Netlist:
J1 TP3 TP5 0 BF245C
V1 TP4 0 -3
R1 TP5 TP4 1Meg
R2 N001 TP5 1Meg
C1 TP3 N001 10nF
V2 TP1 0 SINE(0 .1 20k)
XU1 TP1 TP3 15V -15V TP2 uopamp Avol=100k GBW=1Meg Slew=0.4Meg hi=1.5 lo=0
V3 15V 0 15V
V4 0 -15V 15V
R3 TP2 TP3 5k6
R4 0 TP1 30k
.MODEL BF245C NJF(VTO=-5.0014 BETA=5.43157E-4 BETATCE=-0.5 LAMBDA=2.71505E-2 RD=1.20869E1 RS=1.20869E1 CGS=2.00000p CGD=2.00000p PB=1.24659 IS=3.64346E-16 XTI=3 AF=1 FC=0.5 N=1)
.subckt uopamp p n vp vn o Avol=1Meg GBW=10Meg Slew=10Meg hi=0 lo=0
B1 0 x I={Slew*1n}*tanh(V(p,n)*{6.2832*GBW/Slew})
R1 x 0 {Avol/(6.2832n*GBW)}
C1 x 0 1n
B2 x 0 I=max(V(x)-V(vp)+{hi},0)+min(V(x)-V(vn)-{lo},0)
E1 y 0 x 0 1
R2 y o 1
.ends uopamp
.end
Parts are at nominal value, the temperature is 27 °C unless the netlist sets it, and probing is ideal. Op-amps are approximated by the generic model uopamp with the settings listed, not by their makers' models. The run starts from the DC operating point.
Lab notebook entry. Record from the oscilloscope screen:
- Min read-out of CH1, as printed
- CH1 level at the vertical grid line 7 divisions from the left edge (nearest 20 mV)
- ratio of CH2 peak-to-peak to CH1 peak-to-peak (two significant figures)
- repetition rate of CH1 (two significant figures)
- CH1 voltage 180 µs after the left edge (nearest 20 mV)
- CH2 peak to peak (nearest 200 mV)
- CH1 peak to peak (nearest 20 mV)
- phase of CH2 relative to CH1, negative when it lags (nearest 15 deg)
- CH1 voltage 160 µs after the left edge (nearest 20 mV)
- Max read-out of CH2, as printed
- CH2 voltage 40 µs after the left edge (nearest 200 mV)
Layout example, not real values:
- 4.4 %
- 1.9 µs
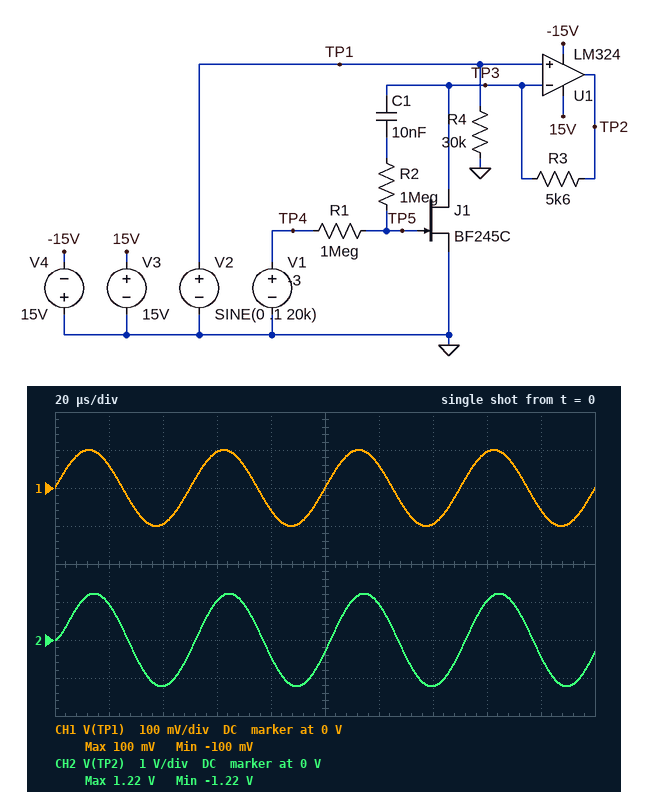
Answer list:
- -100 mV
- -100 mV
- 12
- 20 kHz
- -60 mV
- 2.4 V
- 200 mV
- -15 deg
- 100 mV
- 1.22 V
- -1.2 V
